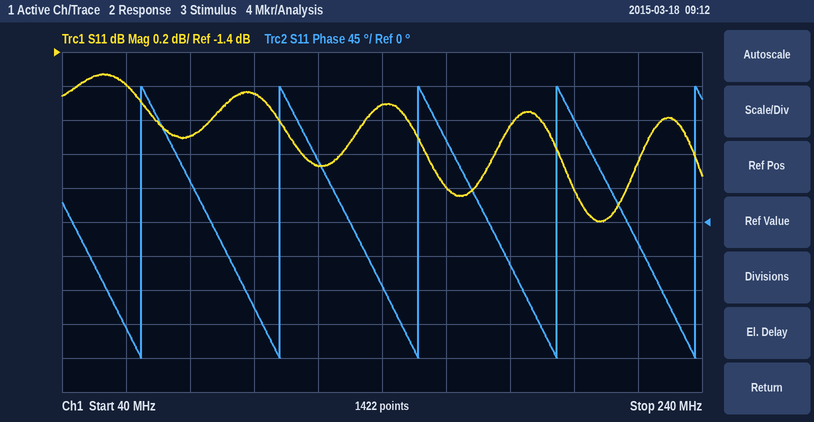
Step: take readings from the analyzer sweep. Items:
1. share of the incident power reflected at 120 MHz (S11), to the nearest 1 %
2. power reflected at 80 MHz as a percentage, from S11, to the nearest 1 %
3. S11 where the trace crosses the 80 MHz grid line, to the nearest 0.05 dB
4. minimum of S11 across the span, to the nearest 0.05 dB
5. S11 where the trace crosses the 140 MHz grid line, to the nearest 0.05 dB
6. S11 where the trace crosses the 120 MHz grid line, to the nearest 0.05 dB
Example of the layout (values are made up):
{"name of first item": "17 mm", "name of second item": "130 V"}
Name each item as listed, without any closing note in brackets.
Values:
{"share of the incident power reflected at 120 MHz (S11), to the nearest 1 %": "62 %", "power reflected at 80 MHz as a percentage, from S11, to the nearest 1 %": "65 %", "S11 where the trace crosses the 80 MHz grid line, to the nearest 0.05 dB": "-1.90 dB", "minimum of S11 across the span, to the nearest 0.05 dB": "-2.40 dB", "S11 where the trace crosses the 140 MHz grid line, to the nearest 0.05 dB": "-1.70 dB", "S11 where the trace crosses the 120 MHz grid line, to the nearest 0.05 dB": "-2.05 dB"}
